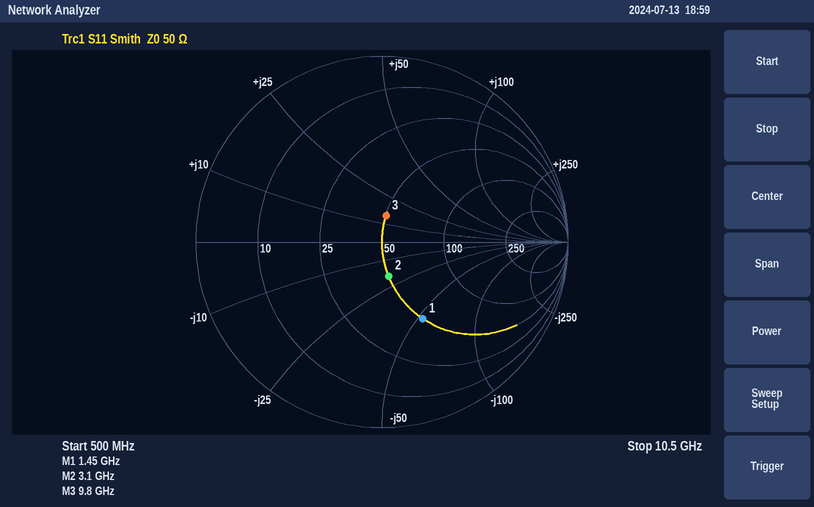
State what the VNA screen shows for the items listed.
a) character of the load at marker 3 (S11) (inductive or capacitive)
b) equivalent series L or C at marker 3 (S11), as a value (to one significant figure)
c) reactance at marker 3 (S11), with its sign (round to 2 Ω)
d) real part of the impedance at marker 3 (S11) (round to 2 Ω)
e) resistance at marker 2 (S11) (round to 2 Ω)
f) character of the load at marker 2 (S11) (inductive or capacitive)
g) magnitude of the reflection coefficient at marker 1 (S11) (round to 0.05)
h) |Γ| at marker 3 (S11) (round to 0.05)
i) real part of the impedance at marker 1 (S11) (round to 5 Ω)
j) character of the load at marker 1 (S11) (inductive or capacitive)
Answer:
inductive
200 pH
+14 Ω
50 Ω
50 Ω
capacitive
0.45
0.15
50 Ω
capacitive
